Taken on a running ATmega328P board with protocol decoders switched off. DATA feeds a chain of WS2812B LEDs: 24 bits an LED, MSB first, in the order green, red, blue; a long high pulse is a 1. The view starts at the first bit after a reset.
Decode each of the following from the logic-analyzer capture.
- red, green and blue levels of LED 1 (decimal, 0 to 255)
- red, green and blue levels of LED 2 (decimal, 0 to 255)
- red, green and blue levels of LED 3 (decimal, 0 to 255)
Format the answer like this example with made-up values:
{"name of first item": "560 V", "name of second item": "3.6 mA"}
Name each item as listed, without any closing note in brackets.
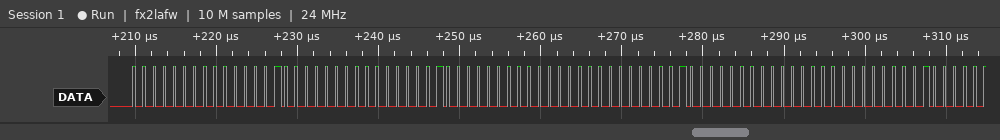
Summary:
{"red, green and blue levels of LED 1": "2, 0, 0", "red, green and blue levels of LED 2": "0, 2, 0", "red, green and blue levels of LED 3": "0, 2, 0"}
